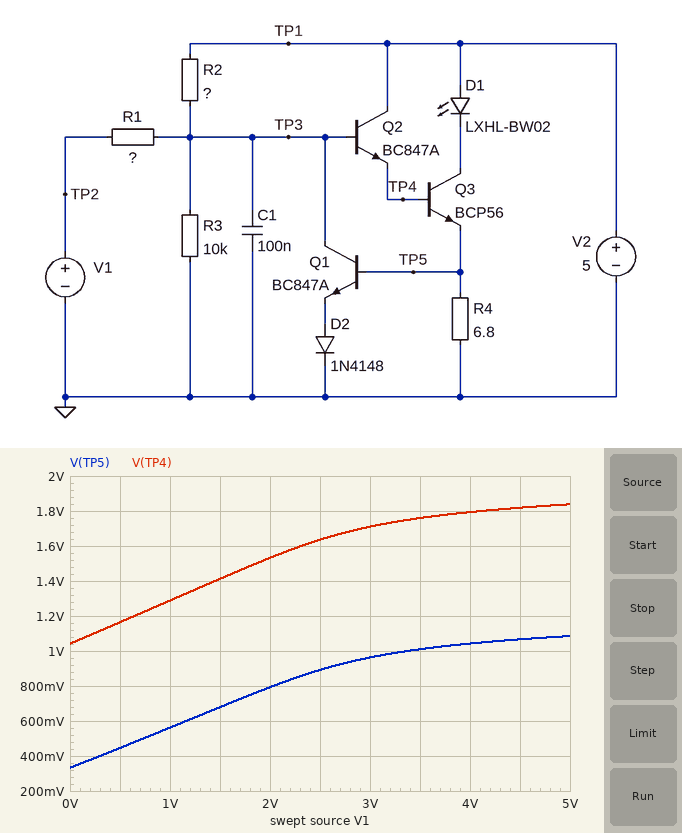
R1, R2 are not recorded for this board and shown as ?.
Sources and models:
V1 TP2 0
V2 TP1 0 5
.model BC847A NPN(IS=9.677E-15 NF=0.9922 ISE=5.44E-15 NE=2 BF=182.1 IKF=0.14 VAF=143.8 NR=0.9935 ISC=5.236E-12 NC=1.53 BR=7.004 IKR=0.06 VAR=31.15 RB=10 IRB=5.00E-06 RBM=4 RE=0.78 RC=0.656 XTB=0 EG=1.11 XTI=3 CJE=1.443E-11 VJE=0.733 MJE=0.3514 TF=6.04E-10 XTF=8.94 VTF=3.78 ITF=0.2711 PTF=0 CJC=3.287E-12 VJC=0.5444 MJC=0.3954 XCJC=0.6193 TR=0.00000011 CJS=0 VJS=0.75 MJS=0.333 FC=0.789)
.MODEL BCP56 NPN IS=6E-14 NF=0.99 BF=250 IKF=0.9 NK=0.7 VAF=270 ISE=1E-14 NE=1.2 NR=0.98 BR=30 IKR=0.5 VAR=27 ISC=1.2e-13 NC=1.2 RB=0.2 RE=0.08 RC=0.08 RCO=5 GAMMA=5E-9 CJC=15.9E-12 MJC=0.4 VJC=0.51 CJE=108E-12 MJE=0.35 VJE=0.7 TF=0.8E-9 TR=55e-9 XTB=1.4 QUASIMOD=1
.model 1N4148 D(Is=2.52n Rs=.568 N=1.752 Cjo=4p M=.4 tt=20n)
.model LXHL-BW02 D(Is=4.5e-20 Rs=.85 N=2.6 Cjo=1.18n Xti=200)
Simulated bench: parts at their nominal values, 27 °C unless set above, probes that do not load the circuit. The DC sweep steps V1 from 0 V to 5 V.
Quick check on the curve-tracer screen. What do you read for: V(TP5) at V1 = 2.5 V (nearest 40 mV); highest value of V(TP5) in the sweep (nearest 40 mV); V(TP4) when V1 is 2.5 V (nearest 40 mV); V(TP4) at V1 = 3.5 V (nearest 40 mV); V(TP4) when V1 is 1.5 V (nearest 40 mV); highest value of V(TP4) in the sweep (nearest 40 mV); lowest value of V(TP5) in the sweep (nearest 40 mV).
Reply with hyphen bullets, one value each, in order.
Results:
- 880 mV
- 1.08 V
- 1.64 V
- 1.76 V
- 1.40 V
- 1.84 V
- 320 mV
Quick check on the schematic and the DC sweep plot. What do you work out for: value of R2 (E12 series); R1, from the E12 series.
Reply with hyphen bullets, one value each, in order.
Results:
- 12 kΩ
- 15 kΩ
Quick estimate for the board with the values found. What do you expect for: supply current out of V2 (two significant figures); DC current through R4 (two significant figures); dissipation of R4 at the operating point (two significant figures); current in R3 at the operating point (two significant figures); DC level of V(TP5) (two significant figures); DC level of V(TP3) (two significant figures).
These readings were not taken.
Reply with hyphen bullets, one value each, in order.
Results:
- 49 mA
- 49 mA
- 16 mW
- 170 µA
- 330 mV
- 1.7 V
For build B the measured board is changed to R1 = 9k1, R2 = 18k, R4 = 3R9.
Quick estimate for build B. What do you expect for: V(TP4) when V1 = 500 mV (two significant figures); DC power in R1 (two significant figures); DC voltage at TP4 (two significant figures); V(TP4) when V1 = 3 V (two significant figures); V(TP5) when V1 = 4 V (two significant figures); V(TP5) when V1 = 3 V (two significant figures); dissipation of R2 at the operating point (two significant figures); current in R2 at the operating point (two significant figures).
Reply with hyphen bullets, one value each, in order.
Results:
- 680 mV
- 120 µW
- 560 mV
- 1.6 V
- 1.0 V
- 810 mV
- 870 µW
- 220 µA
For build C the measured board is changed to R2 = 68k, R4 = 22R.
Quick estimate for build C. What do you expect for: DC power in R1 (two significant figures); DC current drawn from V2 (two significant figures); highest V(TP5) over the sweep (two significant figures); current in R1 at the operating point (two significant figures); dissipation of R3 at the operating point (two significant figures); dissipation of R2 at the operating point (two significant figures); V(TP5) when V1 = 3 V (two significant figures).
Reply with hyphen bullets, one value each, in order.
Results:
- 11 µW
- 68 µA
- 880 mV
- 27 µA
- 16 µW
- 310 µW
- 260 mV
